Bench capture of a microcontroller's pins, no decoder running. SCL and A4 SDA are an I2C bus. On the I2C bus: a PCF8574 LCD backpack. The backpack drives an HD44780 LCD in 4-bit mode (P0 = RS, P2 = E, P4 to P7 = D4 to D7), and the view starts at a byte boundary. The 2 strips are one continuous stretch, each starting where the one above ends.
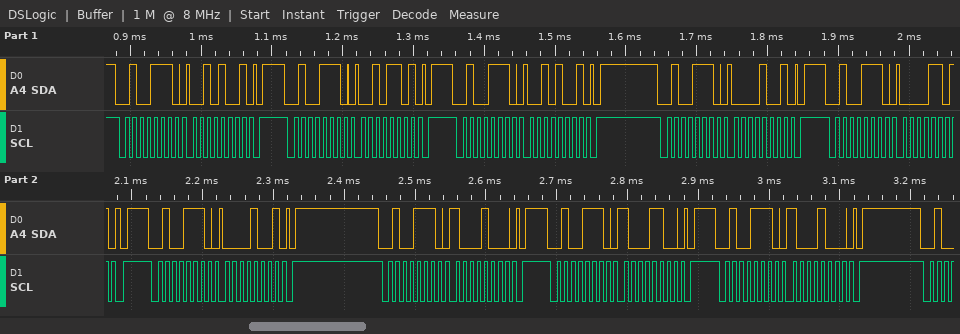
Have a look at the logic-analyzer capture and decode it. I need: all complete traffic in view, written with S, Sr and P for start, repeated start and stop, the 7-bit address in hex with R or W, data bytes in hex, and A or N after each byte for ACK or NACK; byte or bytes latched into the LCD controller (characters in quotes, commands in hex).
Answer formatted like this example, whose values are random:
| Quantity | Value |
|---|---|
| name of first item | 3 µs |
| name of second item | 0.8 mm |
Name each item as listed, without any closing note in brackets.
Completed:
| Quantity | Value |
|---|---|
| all complete traffic in view, written with S, Sr and P for start, repeated start and stop, the 7-bit address in hex with R or W, data bytes in hex, and A or N after each byte for ACK or NACK | S 27W A 29 A P S 27W A 2D A P S 27W A 29 A P S 27W A 09 A P S 27W A 0D A P S 27W A 09 A P S 27W A 88 A P S 27W A 8C A P S 27W A 88 A P |
| byte or bytes latched into the LCD controller | ' ' |
